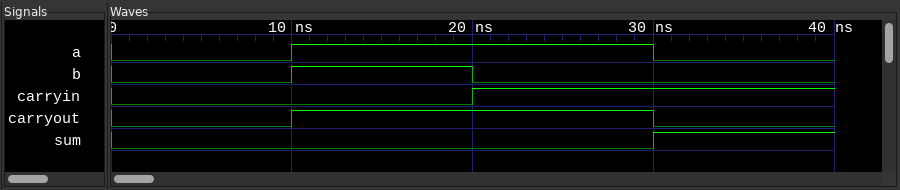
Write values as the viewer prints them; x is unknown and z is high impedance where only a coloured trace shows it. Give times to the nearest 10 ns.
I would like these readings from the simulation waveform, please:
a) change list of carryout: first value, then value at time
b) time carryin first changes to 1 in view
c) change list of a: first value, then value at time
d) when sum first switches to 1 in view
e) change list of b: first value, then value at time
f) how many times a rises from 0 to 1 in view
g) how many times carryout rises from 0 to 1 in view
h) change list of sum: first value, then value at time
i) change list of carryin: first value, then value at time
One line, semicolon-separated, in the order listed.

0, 1 at 10 ns, 0 at 30 ns; 20 ns; 0, 1 at 10 ns, 0 at 30 ns; 30 ns; 0, 1 at 10 ns, 0 at 20 ns; 1; 1; 0, 1 at 30 ns; 0, 1 at 20 ns
